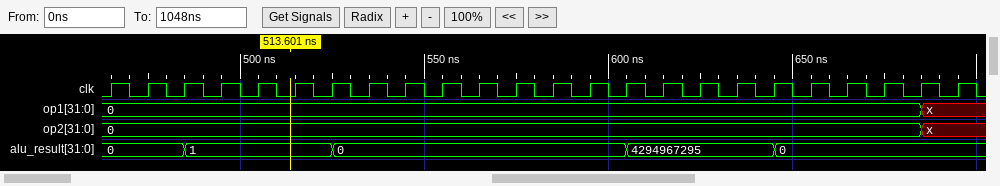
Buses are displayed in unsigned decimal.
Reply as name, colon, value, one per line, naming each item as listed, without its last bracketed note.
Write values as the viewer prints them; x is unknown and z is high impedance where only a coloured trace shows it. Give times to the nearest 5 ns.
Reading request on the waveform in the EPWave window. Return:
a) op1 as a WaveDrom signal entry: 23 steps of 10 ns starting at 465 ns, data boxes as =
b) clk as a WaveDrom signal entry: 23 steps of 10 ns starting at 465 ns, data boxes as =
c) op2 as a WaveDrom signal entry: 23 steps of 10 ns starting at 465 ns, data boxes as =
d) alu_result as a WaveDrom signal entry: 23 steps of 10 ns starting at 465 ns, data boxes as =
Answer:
op1 as a WaveDrom signal entry: 23 steps of 10 ns starting at 465 ns, data boxes as =: {name: 'op1', wave: '=.....................x', data: '0'}
clk as a WaveDrom signal entry: 23 steps of 10 ns starting at 465 ns, data boxes as =: {name: 'clk', wave: 'p......................'}
op2 as a WaveDrom signal entry: 23 steps of 10 ns starting at 465 ns, data boxes as =: {name: 'op2', wave: '=.....................x', data: '0'}
alu_result as a WaveDrom signal entry: 23 steps of 10 ns starting at 465 ns, data boxes as =: {name: 'alu_result', wave: '=.=...=.......=...=....', data: '0 1 0 4294967295 0'}
